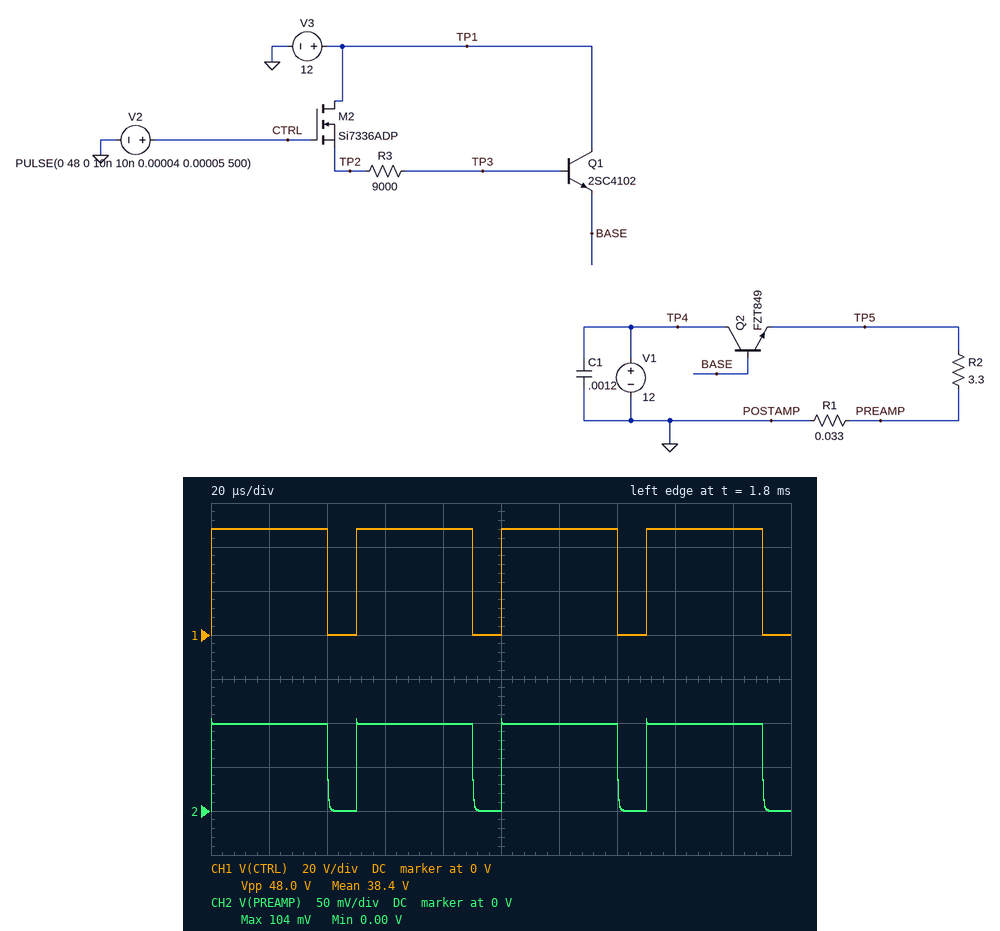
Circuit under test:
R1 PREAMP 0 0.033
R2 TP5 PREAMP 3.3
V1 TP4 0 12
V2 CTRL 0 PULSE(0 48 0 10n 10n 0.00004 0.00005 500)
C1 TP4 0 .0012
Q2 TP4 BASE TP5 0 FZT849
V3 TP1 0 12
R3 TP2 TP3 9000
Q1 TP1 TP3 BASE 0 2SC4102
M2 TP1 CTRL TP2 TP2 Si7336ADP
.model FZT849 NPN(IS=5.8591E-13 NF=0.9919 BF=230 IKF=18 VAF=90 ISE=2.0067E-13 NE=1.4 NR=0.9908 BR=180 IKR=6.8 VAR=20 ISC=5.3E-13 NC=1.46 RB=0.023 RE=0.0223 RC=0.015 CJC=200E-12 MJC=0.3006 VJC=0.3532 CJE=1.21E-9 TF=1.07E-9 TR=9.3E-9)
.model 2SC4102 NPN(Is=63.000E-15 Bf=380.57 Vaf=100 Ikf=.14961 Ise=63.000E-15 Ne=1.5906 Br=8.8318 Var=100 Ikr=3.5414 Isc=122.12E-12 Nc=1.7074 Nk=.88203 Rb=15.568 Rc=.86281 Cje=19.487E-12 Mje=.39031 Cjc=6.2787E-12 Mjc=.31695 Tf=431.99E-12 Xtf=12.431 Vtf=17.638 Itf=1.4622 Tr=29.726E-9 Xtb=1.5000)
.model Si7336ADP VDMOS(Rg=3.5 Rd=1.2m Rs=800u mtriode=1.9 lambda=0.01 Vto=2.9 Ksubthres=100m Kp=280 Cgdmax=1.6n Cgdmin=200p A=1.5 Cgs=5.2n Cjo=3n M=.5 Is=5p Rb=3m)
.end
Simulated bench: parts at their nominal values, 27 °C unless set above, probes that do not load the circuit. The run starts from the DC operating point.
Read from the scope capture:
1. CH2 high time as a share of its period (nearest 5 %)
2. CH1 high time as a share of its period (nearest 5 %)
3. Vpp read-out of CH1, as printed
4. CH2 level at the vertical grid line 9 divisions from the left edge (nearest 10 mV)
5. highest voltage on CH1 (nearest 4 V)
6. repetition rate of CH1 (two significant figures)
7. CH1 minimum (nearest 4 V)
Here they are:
80 %
80 %
48.0 V
100 mV
48 V
20 kHz
0 V
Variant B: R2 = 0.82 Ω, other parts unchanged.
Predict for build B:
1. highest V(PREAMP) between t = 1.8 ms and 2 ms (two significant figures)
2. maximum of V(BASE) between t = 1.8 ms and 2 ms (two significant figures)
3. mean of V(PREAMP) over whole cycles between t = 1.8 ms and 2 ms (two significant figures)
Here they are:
280 mV
8.3 V
230 mV
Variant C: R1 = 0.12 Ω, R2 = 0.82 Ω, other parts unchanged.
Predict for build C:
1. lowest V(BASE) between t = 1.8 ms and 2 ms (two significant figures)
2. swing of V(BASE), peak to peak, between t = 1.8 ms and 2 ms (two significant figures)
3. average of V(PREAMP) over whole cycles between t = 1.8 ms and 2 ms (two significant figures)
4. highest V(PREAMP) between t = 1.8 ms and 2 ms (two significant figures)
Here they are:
550 mV
8.1 V
790 mV
980 mV
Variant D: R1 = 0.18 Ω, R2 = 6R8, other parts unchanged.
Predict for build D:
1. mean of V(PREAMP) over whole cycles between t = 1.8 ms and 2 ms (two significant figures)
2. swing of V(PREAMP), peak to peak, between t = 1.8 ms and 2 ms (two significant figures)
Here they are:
220 mV
280 mV
